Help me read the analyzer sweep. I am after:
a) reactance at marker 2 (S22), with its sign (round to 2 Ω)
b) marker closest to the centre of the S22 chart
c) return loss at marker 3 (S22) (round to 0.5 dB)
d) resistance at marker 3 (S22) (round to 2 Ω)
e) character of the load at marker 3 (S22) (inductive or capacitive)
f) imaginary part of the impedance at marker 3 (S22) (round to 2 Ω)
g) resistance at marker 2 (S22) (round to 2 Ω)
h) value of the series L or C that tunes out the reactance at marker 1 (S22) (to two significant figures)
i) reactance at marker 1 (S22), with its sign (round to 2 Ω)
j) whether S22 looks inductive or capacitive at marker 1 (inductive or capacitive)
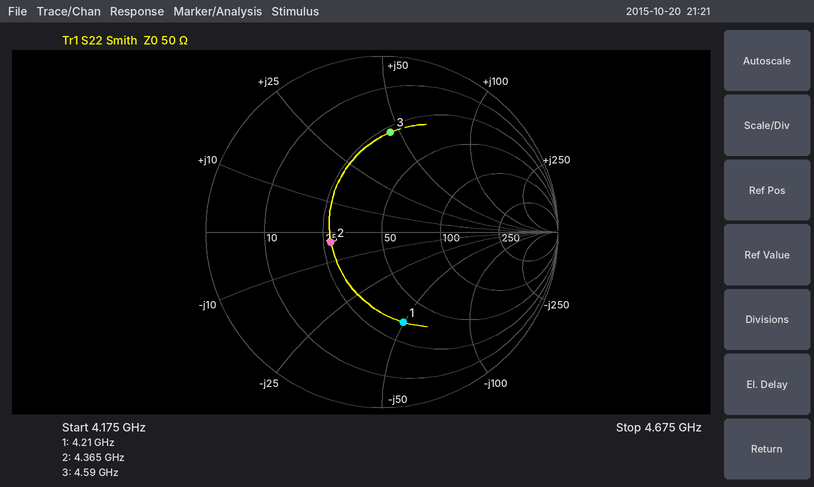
-4 Ω
marker 2
5.0 dB
28 Ω
inductive
+46 Ω
28 Ω
1.9 nH
-50 Ω
capacitive
